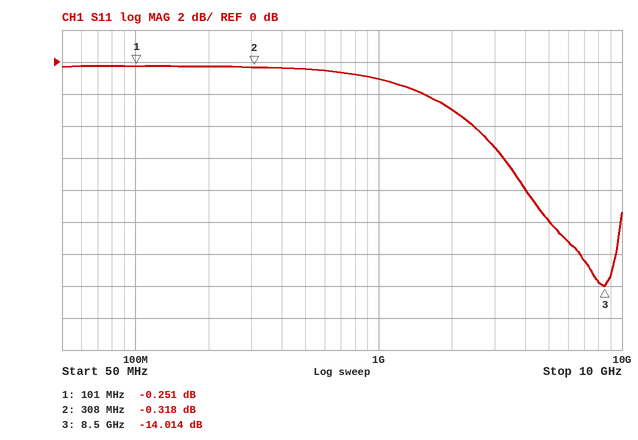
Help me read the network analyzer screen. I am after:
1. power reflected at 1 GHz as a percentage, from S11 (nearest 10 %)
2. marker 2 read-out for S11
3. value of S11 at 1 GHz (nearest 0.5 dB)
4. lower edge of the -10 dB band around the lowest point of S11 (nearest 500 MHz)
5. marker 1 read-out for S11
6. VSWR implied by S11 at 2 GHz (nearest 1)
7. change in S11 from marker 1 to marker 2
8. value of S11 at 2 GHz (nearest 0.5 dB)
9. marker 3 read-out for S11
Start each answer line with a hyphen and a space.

- 80 %
- -0.318 dB
- -1.0 dB
- 5.0 GHz
- -0.251 dB
- 6
- -0.067 dB
- -3.0 dB
- -14.014 dB
